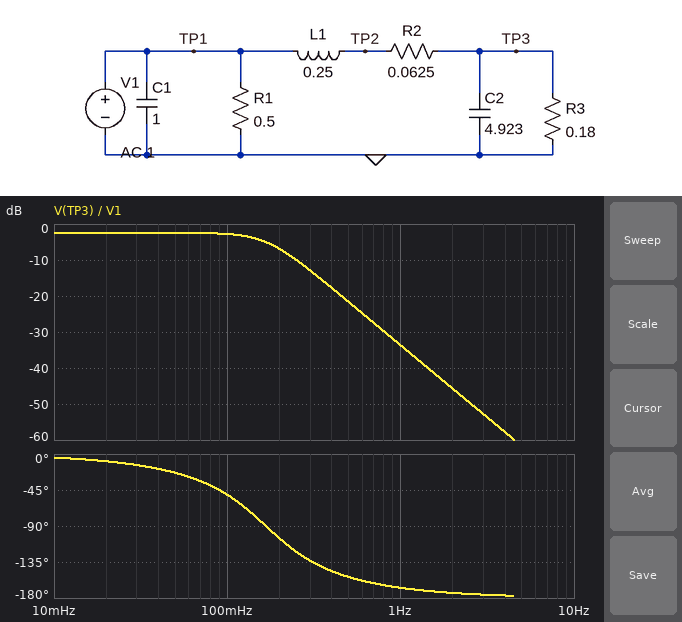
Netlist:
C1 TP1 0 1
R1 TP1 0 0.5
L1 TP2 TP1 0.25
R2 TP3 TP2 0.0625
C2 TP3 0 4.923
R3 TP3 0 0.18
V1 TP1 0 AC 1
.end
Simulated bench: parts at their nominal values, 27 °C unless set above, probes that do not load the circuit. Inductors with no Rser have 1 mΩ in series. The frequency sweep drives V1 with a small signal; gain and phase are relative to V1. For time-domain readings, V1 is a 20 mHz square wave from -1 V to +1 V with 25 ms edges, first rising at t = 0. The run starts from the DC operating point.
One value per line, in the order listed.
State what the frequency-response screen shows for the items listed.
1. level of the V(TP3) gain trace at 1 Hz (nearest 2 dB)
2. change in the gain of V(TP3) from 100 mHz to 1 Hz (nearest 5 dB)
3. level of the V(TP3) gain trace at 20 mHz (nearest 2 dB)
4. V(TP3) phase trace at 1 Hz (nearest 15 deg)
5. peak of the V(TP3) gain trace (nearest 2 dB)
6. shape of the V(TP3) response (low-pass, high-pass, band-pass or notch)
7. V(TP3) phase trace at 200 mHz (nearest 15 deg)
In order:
-34 dB
-30 dB
-2 dB
-165 deg
-2 dB
low-pass
-105 deg
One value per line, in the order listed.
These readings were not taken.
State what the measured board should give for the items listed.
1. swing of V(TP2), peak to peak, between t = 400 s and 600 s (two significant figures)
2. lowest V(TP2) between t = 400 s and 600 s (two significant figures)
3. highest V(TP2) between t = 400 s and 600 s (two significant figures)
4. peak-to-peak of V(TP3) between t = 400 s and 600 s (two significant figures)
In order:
2.3 V
-1.1 V
1.1 V
1.7 V
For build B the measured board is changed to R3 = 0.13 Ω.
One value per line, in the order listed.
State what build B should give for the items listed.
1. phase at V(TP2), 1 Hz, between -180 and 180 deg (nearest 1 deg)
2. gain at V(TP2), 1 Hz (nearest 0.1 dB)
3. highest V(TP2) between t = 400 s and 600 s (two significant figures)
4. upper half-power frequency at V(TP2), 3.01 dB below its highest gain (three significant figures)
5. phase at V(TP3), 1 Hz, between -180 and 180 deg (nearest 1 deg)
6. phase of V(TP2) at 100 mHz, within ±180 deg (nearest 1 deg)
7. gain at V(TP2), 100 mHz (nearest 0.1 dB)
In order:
-111 deg
-26.1 dB
1.0 V
150 mHz
-163 deg
-47 deg
-1.3 dB
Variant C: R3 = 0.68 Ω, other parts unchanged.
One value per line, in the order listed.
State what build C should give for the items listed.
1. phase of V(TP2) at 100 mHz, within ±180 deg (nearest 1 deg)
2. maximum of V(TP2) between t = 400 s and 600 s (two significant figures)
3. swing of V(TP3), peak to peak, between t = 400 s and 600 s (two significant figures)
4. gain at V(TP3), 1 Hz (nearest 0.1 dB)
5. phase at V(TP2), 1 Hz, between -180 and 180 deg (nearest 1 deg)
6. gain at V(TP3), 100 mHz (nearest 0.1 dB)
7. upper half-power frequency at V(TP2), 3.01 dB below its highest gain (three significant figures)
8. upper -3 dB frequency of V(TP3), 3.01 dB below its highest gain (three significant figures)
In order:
-25 deg
1.8 V
3.2 V
-33.6 dB
-114 deg
2.6 dB
178 mHz
177 mHz
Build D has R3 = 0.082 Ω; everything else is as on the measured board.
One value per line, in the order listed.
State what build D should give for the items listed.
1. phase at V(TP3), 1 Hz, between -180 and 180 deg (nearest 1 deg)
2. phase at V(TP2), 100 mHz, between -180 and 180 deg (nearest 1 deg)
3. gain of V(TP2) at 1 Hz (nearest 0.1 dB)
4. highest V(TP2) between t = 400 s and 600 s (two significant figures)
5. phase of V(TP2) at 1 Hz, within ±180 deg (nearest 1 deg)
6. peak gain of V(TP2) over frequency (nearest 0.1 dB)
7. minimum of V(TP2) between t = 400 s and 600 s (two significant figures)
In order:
-156 deg
-52 deg
-25.9 dB
990 mV
-108 deg
-0.1 dB
-990 mV
